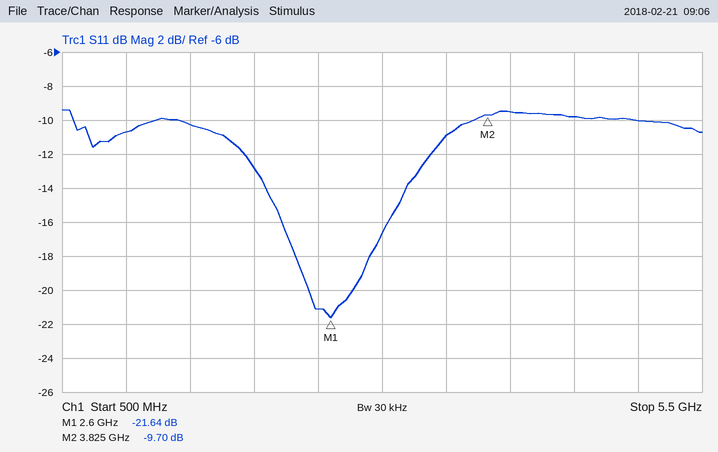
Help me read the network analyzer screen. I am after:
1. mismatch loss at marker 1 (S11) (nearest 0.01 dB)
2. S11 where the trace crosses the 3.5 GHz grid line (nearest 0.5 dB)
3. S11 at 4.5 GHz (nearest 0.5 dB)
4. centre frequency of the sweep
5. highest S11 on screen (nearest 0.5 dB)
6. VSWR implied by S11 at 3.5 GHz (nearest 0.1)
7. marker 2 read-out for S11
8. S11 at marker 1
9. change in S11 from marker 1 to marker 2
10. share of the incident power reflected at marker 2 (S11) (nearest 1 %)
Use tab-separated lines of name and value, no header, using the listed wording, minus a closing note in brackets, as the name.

mismatch loss at marker 1 (S11)	0.03 dB
S11 where the trace crosses the 3.5 GHz grid line	-11.0 dB
S11 at 4.5 GHz	-10.0 dB
centre frequency of the sweep	3 GHz
highest S11 on screen	-9.5 dB
VSWR implied by S11 at 3.5 GHz	1.8
marker 2 read-out for S11	-9.70 dB
S11 at marker 1	-21.64 dB
change in S11 from marker 1 to marker 2	11.94 dB
share of the incident power reflected at marker 2 (S11)	11 %
